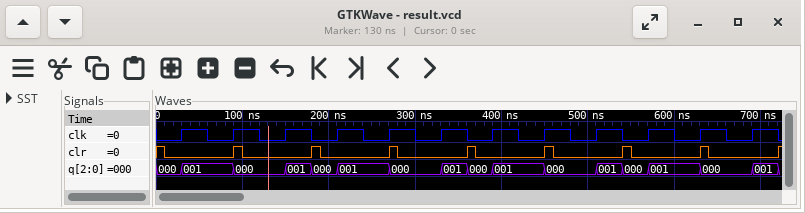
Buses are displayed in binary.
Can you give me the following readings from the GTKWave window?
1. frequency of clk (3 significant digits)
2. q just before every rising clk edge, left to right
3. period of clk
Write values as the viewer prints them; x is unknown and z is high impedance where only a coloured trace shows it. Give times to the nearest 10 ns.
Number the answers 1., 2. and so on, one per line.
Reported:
1. 16.7 MHz
2. 000, 001, 000, 000, 001, 000, 000, 001, 000, 000, 001, 000
3. 60 ns
